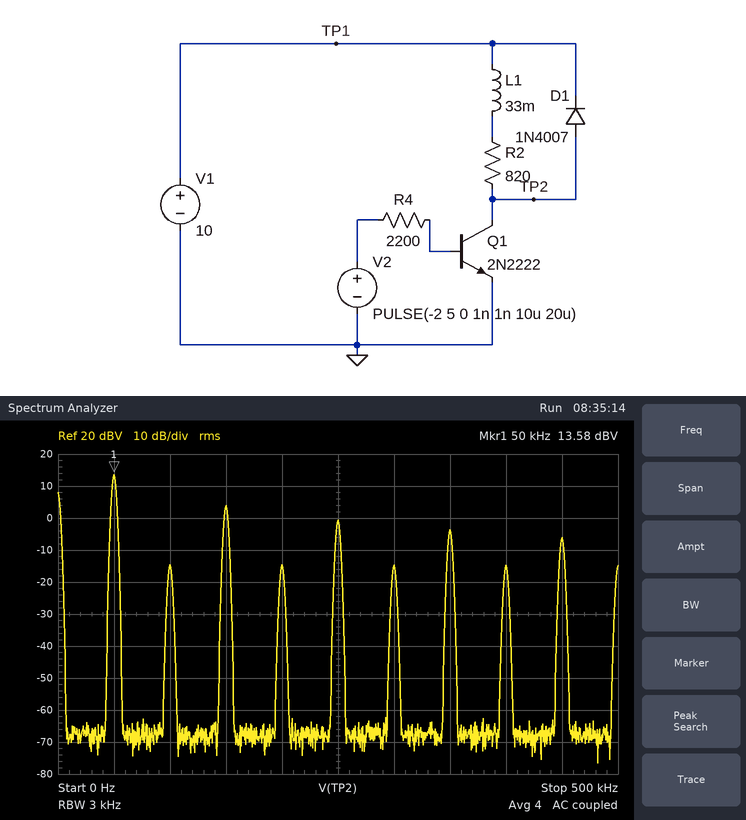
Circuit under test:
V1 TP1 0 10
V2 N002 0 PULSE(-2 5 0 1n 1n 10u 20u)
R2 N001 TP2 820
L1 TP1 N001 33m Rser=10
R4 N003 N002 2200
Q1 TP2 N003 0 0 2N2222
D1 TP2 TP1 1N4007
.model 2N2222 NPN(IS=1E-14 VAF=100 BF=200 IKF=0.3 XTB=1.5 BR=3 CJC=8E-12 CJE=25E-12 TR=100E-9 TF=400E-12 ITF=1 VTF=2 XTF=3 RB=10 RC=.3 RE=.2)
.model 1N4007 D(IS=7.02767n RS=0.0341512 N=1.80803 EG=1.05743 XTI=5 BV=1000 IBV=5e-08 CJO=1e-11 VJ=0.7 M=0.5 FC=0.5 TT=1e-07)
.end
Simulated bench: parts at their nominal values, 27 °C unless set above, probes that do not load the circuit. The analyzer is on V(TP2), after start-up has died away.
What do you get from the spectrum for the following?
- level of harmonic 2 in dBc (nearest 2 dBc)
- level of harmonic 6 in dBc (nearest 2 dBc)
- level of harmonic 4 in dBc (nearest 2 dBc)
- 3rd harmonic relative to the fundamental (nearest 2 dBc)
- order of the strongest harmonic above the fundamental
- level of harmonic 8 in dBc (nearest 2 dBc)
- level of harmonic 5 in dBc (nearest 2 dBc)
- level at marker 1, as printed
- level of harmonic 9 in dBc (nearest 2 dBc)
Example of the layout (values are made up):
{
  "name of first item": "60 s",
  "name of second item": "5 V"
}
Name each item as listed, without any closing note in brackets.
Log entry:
{
  "level of harmonic 2 in dBc": "-28 dBc",
  "level of harmonic 6 in dBc": "-28 dBc",
  "level of harmonic 4 in dBc": "-28 dBc",
  "3rd harmonic relative to the fundamental": "-10 dBc",
  "order of the strongest harmonic above the fundamental": "3",
  "level of harmonic 8 in dBc": "-28 dBc",
  "level of harmonic 5 in dBc": "-14 dBc",
  "level at marker 1, as printed": "13.58 dBV",
  "level of harmonic 9 in dBc": "-20 dBc"
}
